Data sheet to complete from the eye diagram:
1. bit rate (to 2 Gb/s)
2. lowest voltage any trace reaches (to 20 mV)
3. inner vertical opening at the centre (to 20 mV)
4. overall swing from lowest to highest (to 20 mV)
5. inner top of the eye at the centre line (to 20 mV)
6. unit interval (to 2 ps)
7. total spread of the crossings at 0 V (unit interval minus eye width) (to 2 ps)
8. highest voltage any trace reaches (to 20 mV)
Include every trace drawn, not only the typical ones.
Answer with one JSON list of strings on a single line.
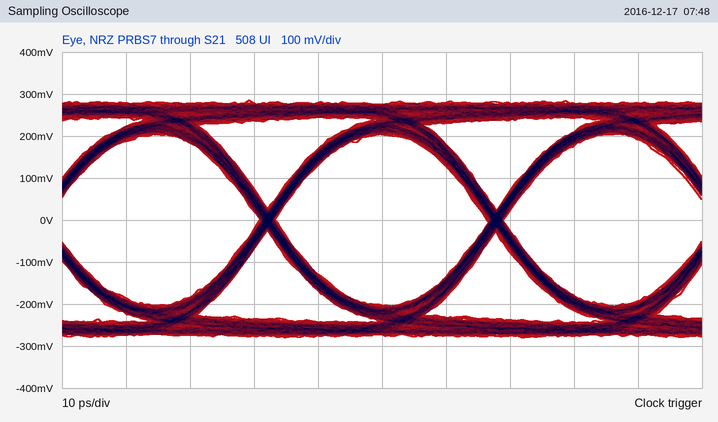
["28 Gb/s", "-280 mV", "400 mV", "560 mV", "200 mV", "36 ps", "2 ps", "280 mV"]
